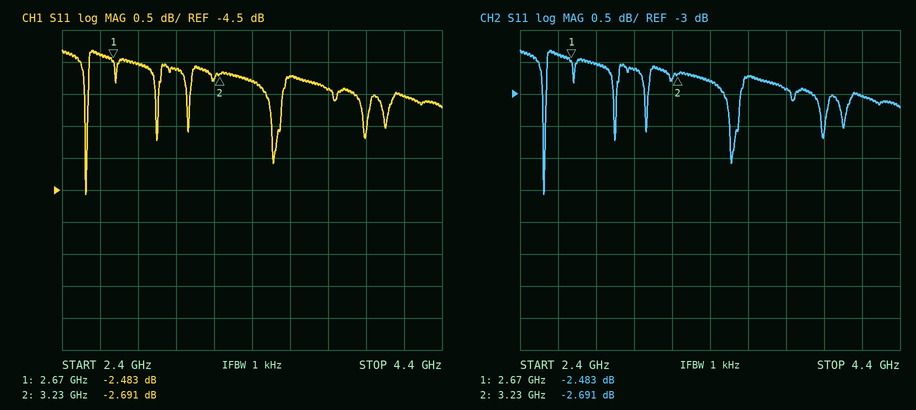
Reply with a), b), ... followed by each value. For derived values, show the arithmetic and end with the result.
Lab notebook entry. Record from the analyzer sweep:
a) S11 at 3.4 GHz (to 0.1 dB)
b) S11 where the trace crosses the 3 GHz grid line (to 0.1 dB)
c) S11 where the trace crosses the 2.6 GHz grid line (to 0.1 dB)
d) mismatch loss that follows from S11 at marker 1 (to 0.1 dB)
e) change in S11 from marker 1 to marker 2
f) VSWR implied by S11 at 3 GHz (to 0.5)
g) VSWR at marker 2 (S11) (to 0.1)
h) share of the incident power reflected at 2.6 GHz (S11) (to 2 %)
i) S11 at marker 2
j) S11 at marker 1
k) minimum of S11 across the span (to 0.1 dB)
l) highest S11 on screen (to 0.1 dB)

a) -2.8 dB
b) -2.6 dB
c) -2.4 dB
d) −10 log10(1 − 10^(-2.483/10)) ≈ 3.6 dB
e) -2.691 − (-2.483) = -0.208 dB
f) |Γ| = 10^(-2.6/20) = 0.7413; VSWR = (1 + 0.7413)/(1 − 0.7413) ≈ 6.73, so 6.5 to the nearest 0.5
g) (1 + 0.7336)/(1 − 0.7336) ≈ 6.5
h) 10^(-2.4/10) ≈ 58 %
i) -2.691 dB
j) -2.483 dB
k) -4.6 dB
l) -2.3 dB
